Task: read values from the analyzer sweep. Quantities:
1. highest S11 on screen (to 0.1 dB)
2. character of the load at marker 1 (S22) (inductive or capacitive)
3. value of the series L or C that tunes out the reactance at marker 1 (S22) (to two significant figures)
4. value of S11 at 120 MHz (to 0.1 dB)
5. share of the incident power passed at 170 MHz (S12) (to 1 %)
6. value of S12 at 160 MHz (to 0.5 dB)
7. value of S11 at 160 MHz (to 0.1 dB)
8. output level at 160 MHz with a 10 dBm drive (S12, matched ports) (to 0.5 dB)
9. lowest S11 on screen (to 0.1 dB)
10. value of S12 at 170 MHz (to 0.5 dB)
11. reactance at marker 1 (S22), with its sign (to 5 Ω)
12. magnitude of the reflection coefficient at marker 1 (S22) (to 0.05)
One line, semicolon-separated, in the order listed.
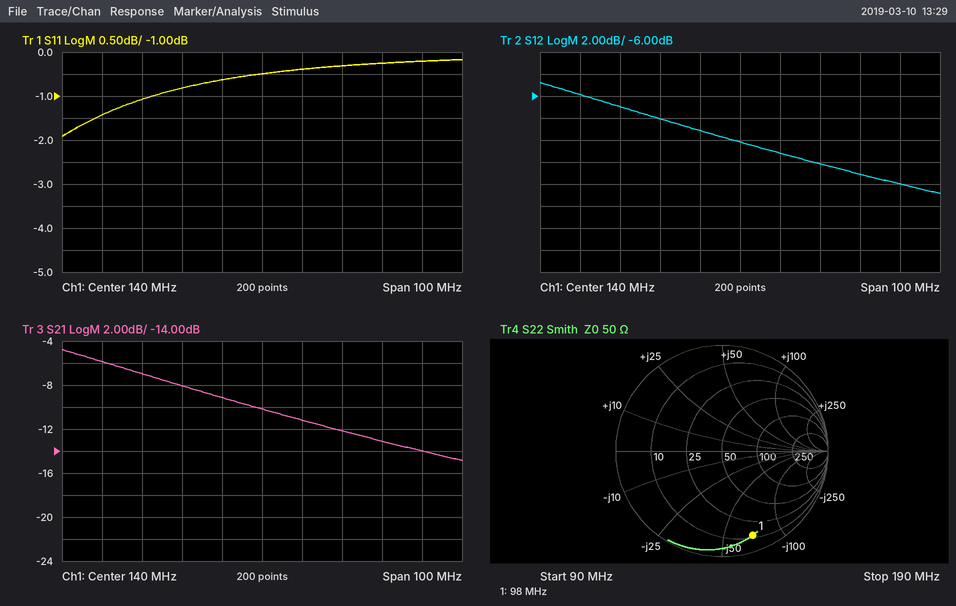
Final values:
-0.2 dB; capacitive; 110 nH; -0.8 dB; 5 %; -12.0 dB; -0.3 dB; -2.0 dBm; -1.9 dB; -13.0 dB; -70 Ω; 0.85
